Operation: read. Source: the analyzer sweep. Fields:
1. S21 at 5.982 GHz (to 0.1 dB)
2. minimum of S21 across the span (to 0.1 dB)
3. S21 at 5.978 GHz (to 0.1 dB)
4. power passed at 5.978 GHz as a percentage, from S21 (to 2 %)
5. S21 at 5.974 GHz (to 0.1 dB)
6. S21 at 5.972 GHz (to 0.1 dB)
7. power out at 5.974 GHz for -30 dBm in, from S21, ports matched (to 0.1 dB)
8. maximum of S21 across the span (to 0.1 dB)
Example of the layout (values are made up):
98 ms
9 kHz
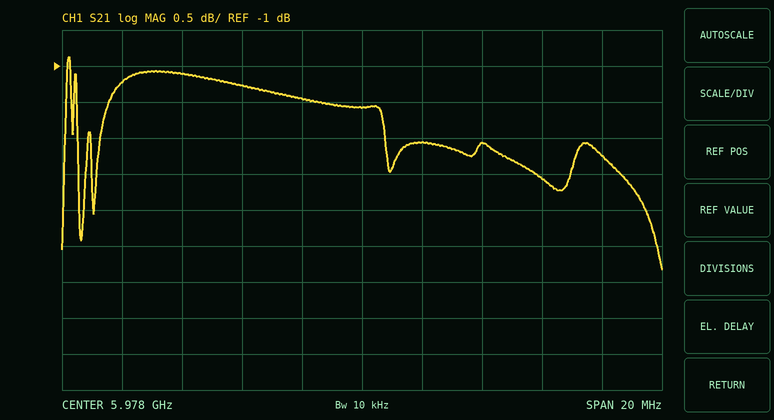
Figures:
-2.1 dB
-3.8 dB
-1.6 dB
70 %
-1.3 dB
-1.1 dB
-31.3 dBm
-0.9 dB
